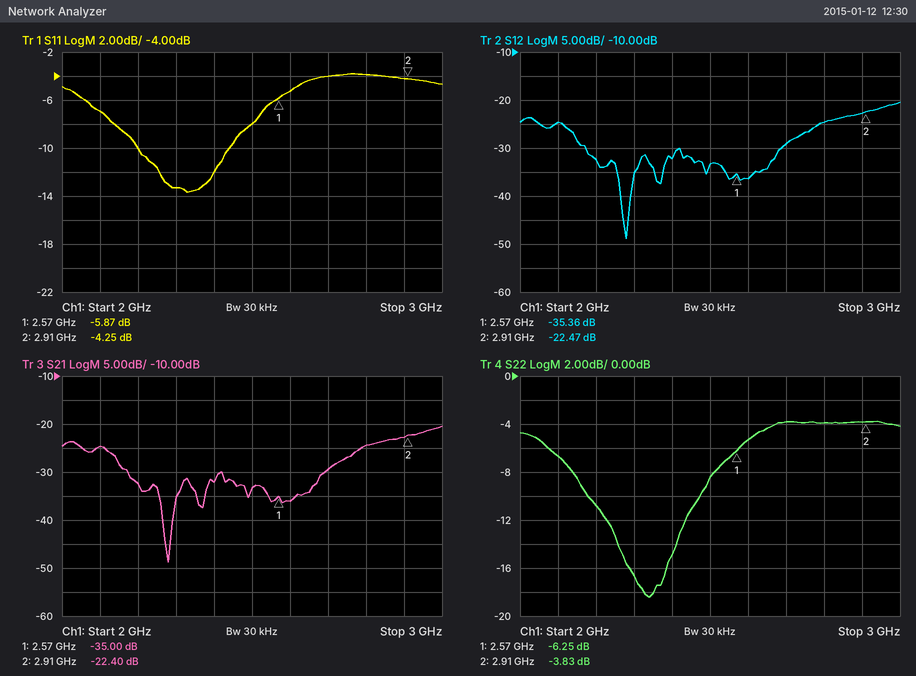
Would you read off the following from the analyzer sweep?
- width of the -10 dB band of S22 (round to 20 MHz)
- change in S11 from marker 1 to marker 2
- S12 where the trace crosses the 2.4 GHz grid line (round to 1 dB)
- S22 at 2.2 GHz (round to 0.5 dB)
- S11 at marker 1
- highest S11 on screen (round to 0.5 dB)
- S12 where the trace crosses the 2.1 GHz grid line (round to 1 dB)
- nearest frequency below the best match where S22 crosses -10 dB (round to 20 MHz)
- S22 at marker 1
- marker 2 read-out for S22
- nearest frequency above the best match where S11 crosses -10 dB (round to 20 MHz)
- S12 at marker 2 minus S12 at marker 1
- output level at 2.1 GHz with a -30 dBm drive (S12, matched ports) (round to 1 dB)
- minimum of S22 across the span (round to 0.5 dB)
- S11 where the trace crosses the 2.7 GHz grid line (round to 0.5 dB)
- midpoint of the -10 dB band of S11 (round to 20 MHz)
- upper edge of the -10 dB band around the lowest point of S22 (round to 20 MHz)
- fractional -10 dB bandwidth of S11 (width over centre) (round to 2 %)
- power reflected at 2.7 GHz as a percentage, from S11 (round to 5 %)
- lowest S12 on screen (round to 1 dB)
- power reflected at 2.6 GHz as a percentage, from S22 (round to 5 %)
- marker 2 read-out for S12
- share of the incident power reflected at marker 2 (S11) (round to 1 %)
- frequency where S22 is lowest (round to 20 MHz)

300 MHz
1.62 dB
-32 dB
-11.0 dB
-5.87 dB
-4.0 dB
-25 dB
2.18 GHz
-6.25 dB
-3.83 dB
2.44 GHz
12.89 dB
-55 dBm
-18.5 dB
-4.0 dB
2.32 GHz
2.48 GHz
10 %
40 %
-49 dB
30 %
-22.47 dB
38 %
2.34 GHz
